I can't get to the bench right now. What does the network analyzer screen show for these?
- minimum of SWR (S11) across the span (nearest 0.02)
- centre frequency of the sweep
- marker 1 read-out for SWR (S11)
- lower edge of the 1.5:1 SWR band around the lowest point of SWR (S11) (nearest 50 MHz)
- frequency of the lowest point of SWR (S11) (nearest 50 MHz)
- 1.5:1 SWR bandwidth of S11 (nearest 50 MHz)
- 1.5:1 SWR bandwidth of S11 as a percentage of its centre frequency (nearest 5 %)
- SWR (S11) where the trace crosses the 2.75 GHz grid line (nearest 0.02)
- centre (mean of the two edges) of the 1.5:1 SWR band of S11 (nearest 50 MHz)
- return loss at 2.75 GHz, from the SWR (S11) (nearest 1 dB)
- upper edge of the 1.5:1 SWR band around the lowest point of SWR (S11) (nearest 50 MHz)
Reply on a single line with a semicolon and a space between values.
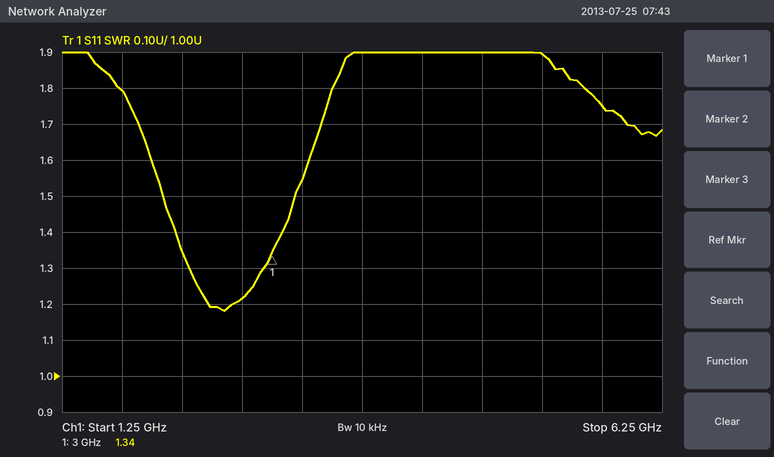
1.18; 3.75 GHz; 1.34; 2.10 GHz; 2.60 GHz; 1.10 GHz; 40 %; 1.22; 2.65 GHz; 20 dB; 3.20 GHz
